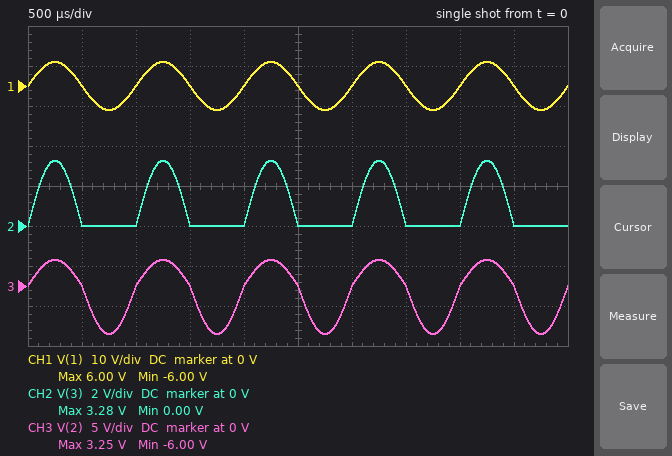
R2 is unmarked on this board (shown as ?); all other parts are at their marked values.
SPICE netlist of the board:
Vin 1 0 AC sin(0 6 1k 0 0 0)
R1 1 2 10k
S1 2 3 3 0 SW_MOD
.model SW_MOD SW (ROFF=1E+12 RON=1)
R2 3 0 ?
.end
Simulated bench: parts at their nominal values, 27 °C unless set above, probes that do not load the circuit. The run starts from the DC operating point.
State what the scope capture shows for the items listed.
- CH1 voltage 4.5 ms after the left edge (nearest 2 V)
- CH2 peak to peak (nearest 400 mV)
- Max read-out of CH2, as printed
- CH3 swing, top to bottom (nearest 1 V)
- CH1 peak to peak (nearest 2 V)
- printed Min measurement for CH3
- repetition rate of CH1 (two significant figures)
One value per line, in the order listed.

0 V
3.2 V
3.28 V
9 V
12 V
-6.00 V
1.0 kHz
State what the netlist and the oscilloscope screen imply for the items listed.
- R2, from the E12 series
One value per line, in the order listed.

12 kΩ
